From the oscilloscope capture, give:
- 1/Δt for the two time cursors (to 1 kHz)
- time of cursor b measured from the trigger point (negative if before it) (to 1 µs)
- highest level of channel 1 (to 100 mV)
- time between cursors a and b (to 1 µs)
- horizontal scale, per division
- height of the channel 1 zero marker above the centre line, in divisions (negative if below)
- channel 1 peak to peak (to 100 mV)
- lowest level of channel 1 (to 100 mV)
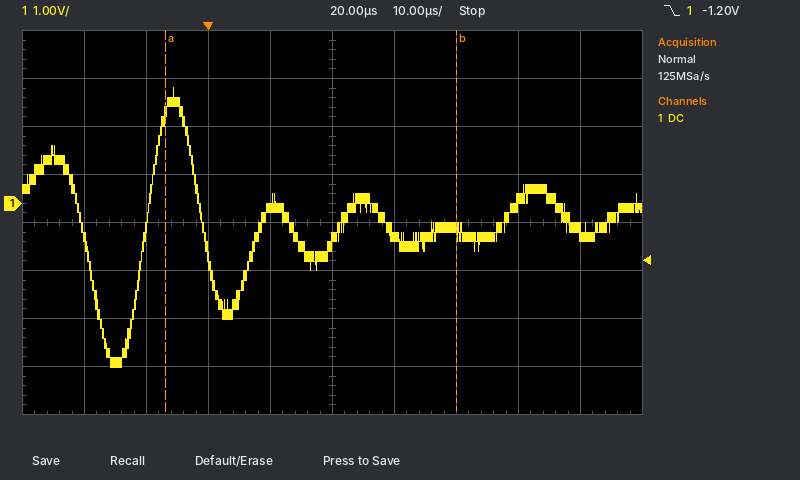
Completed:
21 kHz
+40 µs
2.4 V
47 µs
10 µs
+0.4 div
5.8 V
-3.4 V
